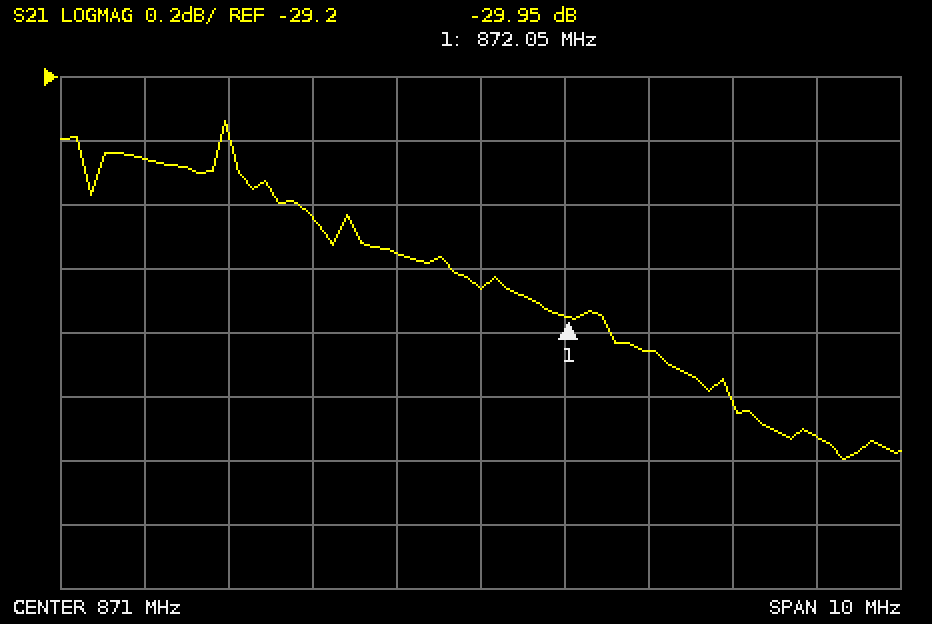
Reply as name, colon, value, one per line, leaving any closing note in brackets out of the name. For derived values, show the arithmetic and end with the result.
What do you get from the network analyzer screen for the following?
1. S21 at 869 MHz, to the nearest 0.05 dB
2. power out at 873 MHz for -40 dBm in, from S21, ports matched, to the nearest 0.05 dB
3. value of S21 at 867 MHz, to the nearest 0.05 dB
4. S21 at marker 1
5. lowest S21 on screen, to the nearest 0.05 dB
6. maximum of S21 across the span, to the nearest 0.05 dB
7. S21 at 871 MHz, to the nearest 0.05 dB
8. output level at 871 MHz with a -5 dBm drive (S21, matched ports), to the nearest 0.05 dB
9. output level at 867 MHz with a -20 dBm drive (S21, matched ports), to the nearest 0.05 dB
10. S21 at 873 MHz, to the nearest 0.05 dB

S21 at 869 MHz, to the nearest 0.05 dB: -29.65 dB
power out at 873 MHz for -40 dBm in, from S21, ports matched, to the nearest 0.05 dB: -40 dBm + (-30.05 dB) = -70.05 dBm
value of S21 at 867 MHz, to the nearest 0.05 dB: -29.45 dB
S21 at marker 1: -29.95 dB
lowest S21 on screen, to the nearest 0.05 dB: -30.40 dB
maximum of S21 across the span, to the nearest 0.05 dB: -29.35 dB
S21 at 871 MHz, to the nearest 0.05 dB: -29.85 dB
output level at 871 MHz with a -5 dBm drive (S21, matched ports), to the nearest 0.05 dB: -5 dBm + (-29.85 dB) = -34.85 dBm
output level at 867 MHz with a -20 dBm drive (S21, matched ports), to the nearest 0.05 dB: -20 dBm + (-29.45 dB) = -49.45 dBm
S21 at 873 MHz, to the nearest 0.05 dB: -30.05 dB
